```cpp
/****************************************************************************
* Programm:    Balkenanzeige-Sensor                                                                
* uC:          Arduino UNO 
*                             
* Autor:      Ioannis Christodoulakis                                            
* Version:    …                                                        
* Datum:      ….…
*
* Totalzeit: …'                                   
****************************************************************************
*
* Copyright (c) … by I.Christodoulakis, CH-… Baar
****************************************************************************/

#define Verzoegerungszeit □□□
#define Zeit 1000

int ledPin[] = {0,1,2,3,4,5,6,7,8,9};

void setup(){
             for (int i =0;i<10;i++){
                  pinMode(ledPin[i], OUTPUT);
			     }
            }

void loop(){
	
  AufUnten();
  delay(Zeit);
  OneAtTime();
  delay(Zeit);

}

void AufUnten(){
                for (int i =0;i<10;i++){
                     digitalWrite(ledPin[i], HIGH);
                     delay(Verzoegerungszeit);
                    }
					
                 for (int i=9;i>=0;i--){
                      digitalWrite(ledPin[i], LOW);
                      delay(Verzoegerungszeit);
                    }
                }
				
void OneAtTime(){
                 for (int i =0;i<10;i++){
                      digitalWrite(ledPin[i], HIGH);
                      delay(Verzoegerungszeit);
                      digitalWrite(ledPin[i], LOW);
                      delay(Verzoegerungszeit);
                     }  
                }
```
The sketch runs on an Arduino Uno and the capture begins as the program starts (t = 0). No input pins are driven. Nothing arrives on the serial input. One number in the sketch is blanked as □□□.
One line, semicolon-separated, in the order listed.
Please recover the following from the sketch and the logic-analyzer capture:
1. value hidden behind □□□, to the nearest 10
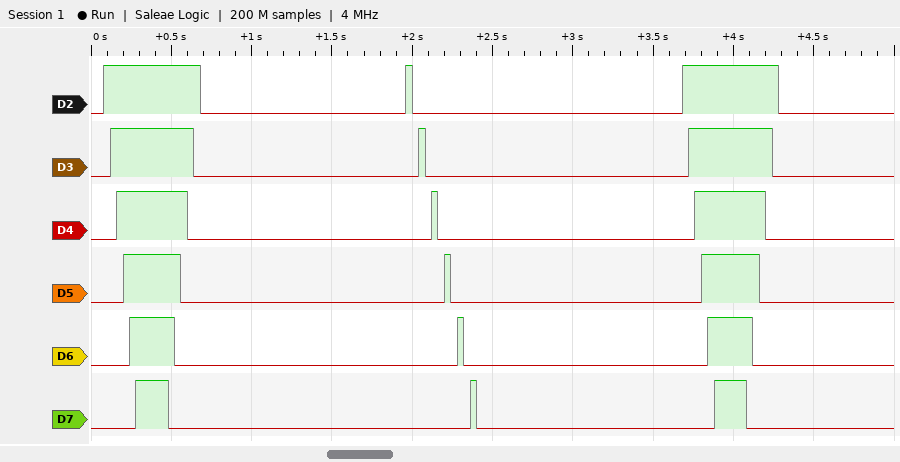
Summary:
40
